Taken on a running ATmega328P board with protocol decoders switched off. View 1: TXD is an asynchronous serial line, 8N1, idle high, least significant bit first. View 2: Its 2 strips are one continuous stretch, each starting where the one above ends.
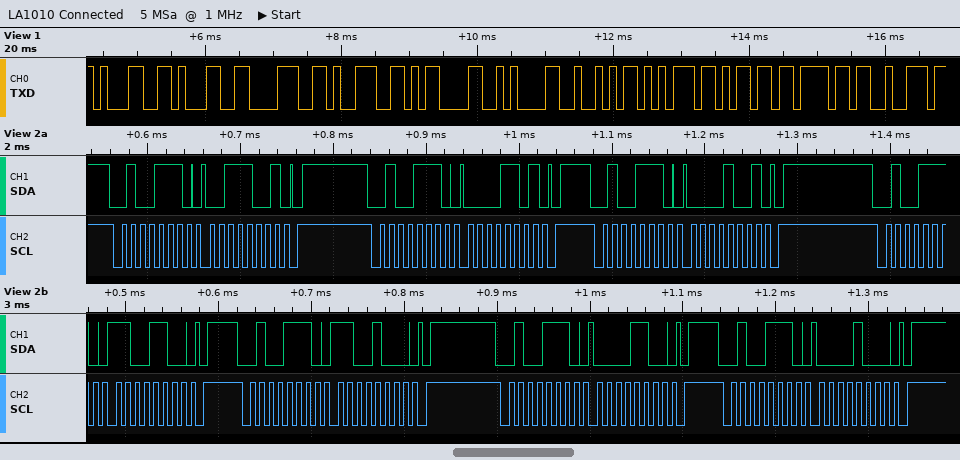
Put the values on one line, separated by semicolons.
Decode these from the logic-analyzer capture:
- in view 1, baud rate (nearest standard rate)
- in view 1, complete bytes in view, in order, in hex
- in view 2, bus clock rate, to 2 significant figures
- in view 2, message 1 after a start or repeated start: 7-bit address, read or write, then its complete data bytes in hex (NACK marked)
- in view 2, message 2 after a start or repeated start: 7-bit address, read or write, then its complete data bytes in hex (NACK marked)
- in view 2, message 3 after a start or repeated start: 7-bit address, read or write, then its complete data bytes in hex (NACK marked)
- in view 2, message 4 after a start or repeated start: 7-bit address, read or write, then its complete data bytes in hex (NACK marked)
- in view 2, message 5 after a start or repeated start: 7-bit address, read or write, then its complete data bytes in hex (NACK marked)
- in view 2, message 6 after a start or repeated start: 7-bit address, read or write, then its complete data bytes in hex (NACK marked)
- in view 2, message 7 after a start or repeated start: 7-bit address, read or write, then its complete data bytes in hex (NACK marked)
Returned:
9600 baud; 31 31 38 39 0D 0A 52 75 6D 6F 72; 100 kHz; 0x27 write: 39; 0x27 write: 0D; 0x27 write: 09; 0x27 write: CC; 0x27 write: C8; 0x27 write: 0C; 0x27 write: 08
